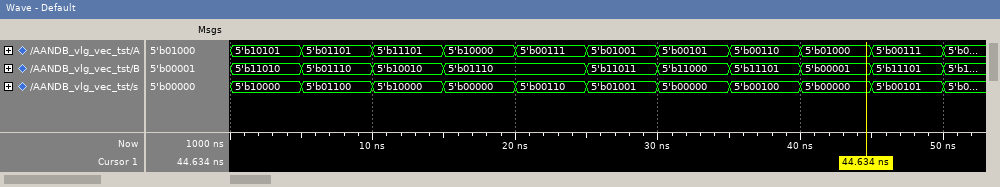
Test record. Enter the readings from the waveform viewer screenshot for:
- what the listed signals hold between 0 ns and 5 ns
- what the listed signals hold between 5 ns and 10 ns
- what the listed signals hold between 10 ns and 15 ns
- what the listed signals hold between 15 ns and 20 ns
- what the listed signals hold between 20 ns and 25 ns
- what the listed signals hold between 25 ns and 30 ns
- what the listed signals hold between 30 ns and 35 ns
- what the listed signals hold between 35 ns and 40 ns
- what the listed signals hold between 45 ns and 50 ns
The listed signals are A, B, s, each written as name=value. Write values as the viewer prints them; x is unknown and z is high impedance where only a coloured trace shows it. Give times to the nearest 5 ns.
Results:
A=5'b10101, B=5'b11010, s=5'b10000
A=5'b01101, B=5'b01110, s=5'b01100
A=5'b11101, B=5'b10010, s=5'b10000
A=5'b10000, B=5'b01110, s=5'b00000
A=5'b00111, B=5'b01110, s=5'b00110
A=5'b01001, B=5'b11011, s=5'b01001
A=5'b00101, B=5'b11000, s=5'b00000
A=5'b00110, B=5'b11101, s=5'b00100
A=5'b00111, B=5'b11101, s=5'b00101
